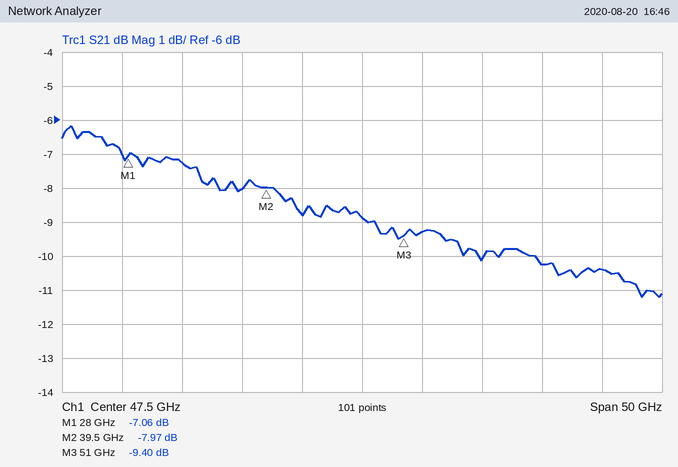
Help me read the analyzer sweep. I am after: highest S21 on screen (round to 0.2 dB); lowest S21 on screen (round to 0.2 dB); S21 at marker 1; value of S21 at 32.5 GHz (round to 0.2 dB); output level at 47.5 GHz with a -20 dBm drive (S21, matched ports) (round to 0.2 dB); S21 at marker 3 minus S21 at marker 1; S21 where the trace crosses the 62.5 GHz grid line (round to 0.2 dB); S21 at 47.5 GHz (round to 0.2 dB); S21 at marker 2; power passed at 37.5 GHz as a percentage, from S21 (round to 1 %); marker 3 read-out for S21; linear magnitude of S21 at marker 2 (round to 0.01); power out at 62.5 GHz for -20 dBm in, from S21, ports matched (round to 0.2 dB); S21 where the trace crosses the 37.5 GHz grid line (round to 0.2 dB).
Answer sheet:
-6.2 dB
-11.2 dB
-7.06 dB
-7.2 dB
-28.8 dBm
-2.34 dB
-10.2 dB
-8.8 dB
-7.97 dB
16 %
-9.40 dB
0.40
-30.2 dBm
-8.0 dB
